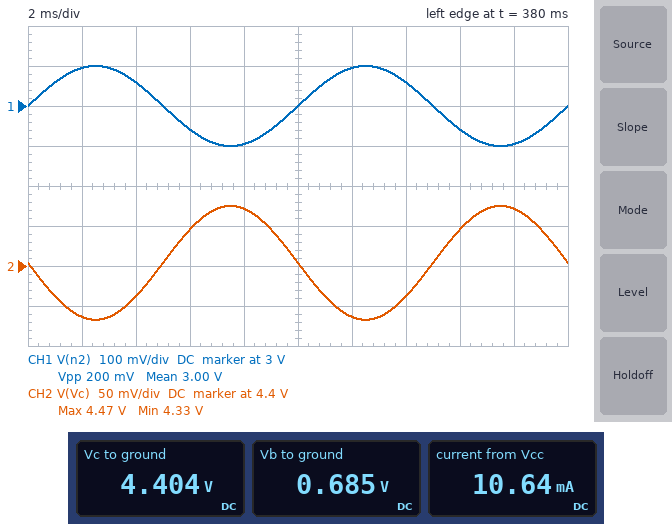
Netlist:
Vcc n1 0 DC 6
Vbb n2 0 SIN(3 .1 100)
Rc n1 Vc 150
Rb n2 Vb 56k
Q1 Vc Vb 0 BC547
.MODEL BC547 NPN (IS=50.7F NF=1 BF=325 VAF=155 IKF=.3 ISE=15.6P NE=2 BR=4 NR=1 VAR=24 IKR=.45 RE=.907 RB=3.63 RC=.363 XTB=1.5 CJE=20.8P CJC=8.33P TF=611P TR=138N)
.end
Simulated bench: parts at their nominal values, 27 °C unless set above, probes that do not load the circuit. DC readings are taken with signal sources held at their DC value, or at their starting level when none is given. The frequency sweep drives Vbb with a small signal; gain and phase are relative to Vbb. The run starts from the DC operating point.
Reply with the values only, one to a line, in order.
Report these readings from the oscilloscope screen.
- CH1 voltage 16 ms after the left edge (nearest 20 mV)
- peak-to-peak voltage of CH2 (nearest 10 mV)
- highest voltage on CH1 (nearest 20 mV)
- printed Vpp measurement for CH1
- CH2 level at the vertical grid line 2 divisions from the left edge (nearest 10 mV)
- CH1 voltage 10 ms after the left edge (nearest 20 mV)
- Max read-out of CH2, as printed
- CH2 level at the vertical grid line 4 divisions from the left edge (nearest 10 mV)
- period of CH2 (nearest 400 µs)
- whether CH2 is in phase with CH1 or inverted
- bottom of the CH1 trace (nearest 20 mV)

2.94 V
140 mV
3.10 V
200 mV
4.36 V
3.00 V
4.47 V
4.47 V
10.0 ms
inverted
2.90 V
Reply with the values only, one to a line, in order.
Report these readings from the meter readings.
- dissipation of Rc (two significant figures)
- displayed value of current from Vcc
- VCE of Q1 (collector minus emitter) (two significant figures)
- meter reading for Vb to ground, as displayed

17 mW
10.64 mA
4.4 V
0.685 V
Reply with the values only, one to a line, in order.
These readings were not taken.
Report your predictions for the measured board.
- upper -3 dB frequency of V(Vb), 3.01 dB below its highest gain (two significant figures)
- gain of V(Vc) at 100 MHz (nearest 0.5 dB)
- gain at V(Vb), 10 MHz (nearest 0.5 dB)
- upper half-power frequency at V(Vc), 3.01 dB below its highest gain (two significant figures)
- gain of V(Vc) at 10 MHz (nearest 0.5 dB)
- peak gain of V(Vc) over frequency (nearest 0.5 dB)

430 kHz
-50.5 dB
-63.0 dB
430 kHz
-30.5 dB
-3.0 dB
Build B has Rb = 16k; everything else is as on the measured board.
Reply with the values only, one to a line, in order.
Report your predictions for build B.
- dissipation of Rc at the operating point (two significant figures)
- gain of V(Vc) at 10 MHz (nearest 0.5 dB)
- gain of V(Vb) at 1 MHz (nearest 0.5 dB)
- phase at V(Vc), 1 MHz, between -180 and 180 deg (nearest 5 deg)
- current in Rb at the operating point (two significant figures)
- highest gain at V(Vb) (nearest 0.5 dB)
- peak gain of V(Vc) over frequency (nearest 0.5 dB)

190 mW
-22.5 dB
-41.5 dB
110 deg
140 µA
-32.0 dB
6.5 dB
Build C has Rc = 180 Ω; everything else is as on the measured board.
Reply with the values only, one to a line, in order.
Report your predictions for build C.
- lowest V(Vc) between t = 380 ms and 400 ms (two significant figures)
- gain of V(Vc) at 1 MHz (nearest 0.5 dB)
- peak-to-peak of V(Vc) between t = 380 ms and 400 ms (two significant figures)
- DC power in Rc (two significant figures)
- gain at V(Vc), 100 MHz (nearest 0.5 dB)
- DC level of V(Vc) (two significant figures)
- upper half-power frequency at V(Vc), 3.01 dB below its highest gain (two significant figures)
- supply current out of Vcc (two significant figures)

4.0 V
-10.5 dB
170 mV
20 mW
-50.0 dB
4.1 V
380 kHz
11 mA
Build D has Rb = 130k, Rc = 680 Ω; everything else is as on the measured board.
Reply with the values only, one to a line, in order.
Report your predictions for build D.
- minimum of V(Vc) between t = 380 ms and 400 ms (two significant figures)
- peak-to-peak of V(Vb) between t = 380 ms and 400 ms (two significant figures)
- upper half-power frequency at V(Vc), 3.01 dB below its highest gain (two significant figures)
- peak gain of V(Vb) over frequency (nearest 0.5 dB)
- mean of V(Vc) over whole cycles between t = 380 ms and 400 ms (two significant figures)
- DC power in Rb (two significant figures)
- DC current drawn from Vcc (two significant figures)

3.0 V
2.9 mV
140 kHz
-37.0 dB
3.1 V
42 µW
4.3 mA
